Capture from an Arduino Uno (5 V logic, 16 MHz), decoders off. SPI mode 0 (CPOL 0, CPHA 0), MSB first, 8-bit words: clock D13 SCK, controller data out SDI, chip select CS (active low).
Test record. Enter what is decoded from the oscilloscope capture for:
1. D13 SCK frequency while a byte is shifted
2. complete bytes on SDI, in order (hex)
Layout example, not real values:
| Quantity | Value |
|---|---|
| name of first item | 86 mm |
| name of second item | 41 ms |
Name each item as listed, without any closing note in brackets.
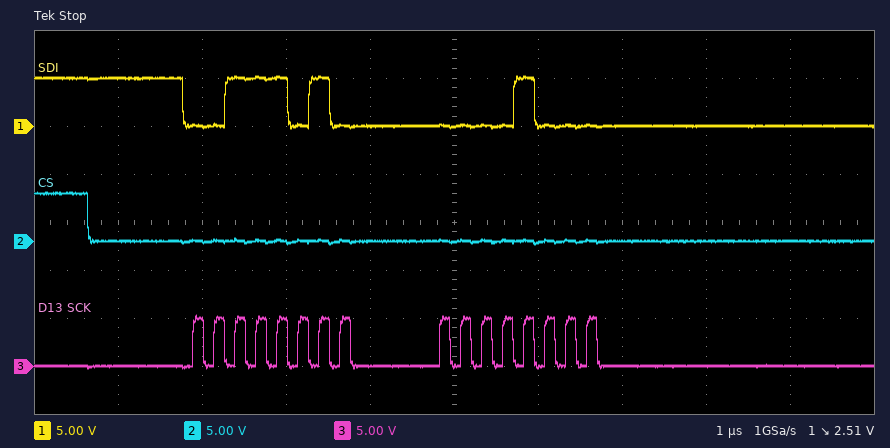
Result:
| Quantity | Value |
|---|---|
| D13 SCK frequency while a byte is shifted | 4 MHz |
| complete bytes on SDI, in order | 3A 08 |
